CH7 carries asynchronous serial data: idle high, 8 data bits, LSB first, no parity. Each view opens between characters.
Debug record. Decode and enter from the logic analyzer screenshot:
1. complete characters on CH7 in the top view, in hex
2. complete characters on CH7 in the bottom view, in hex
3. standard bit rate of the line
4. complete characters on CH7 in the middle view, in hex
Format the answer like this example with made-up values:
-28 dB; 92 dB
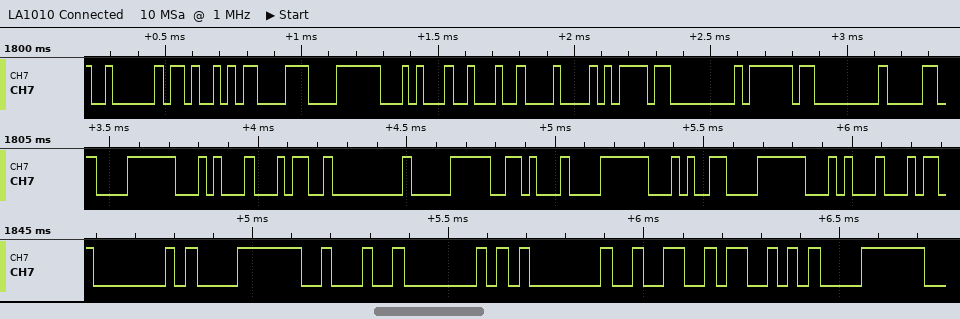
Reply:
02, 4B, C3, F8, 14, 22, 08, BD, 00, BF, 00; 40, F8, 22, 40, 01, 32, 53, F8; 38400 baud; F8, 14, 34, 00, F0, 16, F8, 94, F8, 14
